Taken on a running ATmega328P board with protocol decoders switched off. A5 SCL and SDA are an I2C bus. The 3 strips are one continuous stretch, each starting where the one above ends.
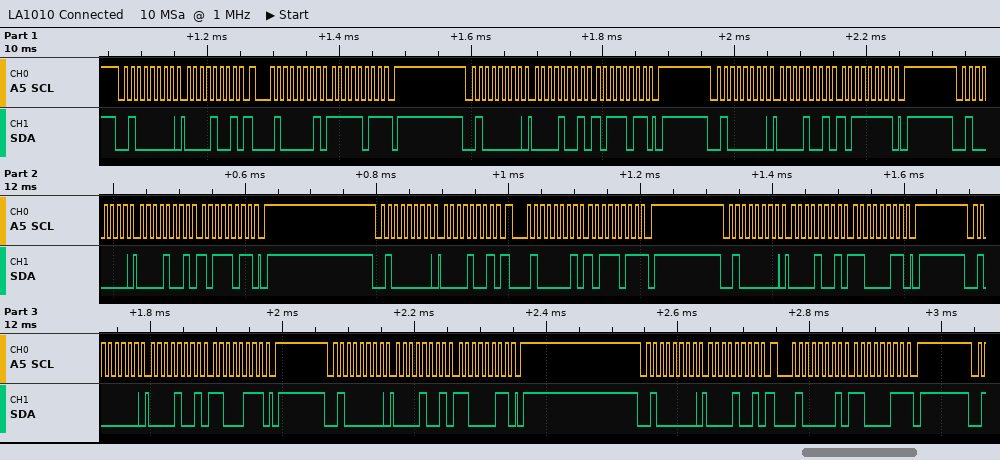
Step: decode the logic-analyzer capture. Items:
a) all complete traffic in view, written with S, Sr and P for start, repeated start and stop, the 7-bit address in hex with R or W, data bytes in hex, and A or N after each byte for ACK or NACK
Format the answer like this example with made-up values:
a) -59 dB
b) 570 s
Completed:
a) S 20W A 09 A Sr 20R A FB N P S 20W A 09 A BB A P S 20W A 09 A BF A P S 20W A 09 A BB A P S 20W A 09 A Sr 20R A BB N P S 20W A 09 A C3 A P S 20W A 09 A C7 A P S 20W A 09 A C3 A P S 20W A 09 A Sr 20R A C3 N P
